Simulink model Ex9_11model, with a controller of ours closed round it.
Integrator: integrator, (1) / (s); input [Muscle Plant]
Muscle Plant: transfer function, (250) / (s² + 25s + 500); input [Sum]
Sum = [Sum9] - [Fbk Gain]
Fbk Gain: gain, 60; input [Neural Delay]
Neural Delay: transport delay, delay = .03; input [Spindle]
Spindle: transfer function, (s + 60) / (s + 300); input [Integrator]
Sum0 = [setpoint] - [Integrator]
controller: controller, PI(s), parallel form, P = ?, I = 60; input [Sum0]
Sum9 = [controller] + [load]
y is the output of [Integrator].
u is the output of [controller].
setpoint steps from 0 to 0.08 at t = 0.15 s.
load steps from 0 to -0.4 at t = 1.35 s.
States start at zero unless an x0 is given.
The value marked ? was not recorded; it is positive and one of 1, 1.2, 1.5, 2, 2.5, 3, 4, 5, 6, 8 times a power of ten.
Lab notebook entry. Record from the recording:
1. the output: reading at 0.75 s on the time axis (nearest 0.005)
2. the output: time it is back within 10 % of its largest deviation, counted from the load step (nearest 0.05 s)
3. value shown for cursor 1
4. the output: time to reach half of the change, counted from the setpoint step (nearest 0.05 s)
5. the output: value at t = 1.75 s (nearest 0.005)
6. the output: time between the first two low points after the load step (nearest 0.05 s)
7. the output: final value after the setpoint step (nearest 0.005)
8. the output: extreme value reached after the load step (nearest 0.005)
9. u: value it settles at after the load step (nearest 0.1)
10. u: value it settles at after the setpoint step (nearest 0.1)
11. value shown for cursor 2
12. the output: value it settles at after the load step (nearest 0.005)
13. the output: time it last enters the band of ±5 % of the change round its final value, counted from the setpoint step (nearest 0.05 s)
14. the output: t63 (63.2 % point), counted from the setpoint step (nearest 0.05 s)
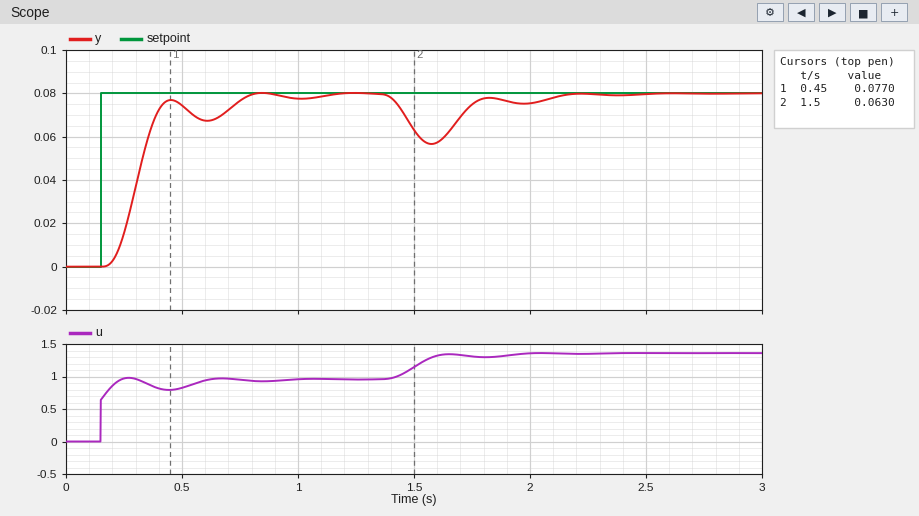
0.075
0.75 s
0.0770
0.15 s
0.075
0.40 s
0.080
0.055
1.4
1.0
0.0630
0.080
0.60 s
0.20 s
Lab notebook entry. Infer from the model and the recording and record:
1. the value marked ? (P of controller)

8
